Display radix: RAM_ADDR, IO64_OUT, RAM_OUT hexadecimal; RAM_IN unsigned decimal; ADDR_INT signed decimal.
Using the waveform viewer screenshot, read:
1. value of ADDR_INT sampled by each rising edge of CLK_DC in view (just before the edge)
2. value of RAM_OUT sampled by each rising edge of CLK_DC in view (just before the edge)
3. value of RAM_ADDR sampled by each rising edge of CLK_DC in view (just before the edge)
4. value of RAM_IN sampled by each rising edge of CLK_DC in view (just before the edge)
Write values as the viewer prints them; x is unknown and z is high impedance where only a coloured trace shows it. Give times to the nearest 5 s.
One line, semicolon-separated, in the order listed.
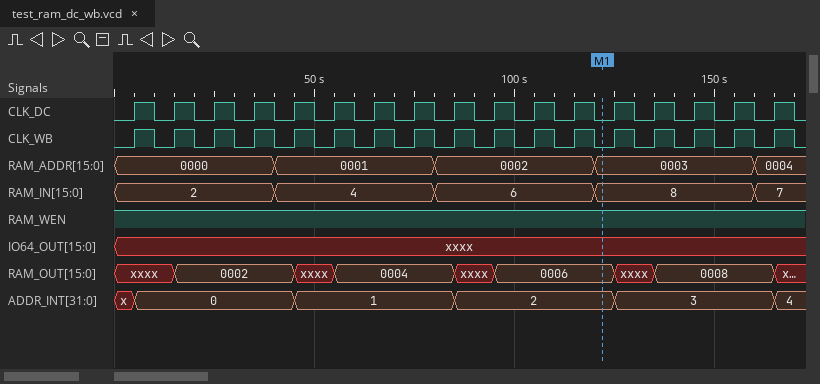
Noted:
x, 0, 0, 0, 0, 1, 1, 1, 1, 2, 2, 2, 2, 3, 3, 3, 3; xxxx, xxxx, 0002, 0002, 0002, xxxx, 0004, 0004, 0004, xxxx, 0006, 0006, 0006, xxxx, 0008, 0008, 0008; 0000, 0000, 0000, 0000, 0001, 0001, 0001, 0001, 0002, 0002, 0002, 0002, 0003, 0003, 0003, 0003, 0004; 2, 2, 2, 2, 4, 4, 4, 4, 6, 6, 6, 6, 8, 8, 8, 8, 7
